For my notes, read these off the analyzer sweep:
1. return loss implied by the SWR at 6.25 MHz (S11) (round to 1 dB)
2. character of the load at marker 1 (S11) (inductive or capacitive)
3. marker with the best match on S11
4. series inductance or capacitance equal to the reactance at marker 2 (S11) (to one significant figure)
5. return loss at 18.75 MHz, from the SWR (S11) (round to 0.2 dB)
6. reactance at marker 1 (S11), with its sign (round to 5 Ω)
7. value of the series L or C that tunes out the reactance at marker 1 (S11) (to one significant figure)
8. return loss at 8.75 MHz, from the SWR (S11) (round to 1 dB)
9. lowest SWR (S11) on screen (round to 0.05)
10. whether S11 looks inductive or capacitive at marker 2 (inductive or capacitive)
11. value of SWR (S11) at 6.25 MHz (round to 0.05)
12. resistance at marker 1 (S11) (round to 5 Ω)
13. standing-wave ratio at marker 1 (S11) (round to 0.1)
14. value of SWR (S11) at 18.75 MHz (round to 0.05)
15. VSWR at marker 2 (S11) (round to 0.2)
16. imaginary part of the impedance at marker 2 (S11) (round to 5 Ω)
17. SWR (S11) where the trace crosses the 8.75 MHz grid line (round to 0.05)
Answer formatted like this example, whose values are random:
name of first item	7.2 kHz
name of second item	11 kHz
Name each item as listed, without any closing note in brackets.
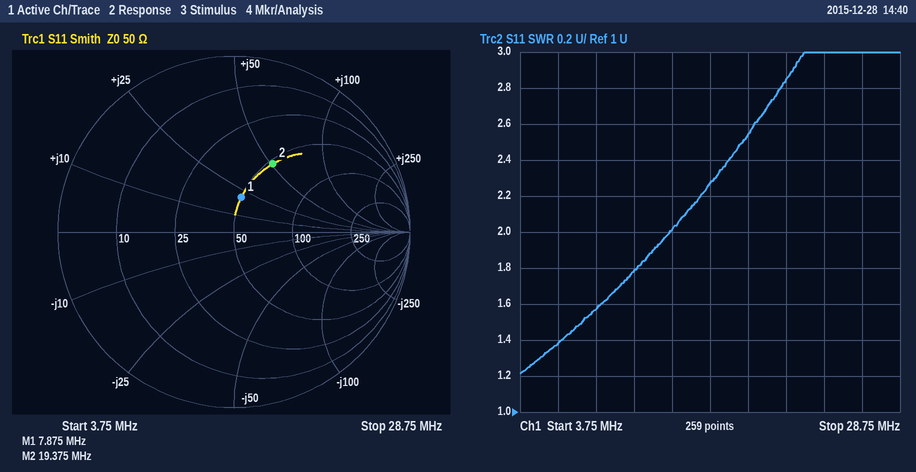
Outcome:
return loss implied by the SWR at 6.25 MHz (S11)	16 dB
character of the load at marker 1 (S11)	inductive
marker with the best match on S11	marker 1
series inductance or capacitance equal to the reactance at marker 2 (S11)	400 nH
return loss at 18.75 MHz, from the SWR (S11)	7.2 dB
reactance at marker 1 (S11), with its sign	+20 Ω
value of the series L or C that tunes out the reactance at marker 1 (S11)	1.0 nF
return loss at 8.75 MHz, from the SWR (S11)	13 dB
lowest SWR (S11) on screen	1.20
whether S11 looks inductive or capacitive at marker 2	inductive
value of SWR (S11) at 6.25 MHz	1.40
resistance at marker 1 (S11)	50 Ω
standing-wave ratio at marker 1 (S11)	1.5
value of SWR (S11) at 18.75 MHz	2.55
VSWR at marker 2 (S11)	2.6
imaginary part of the impedance at marker 2 (S11)	+50 Ω
SWR (S11) where the trace crosses the 8.75 MHz grid line	1.55
